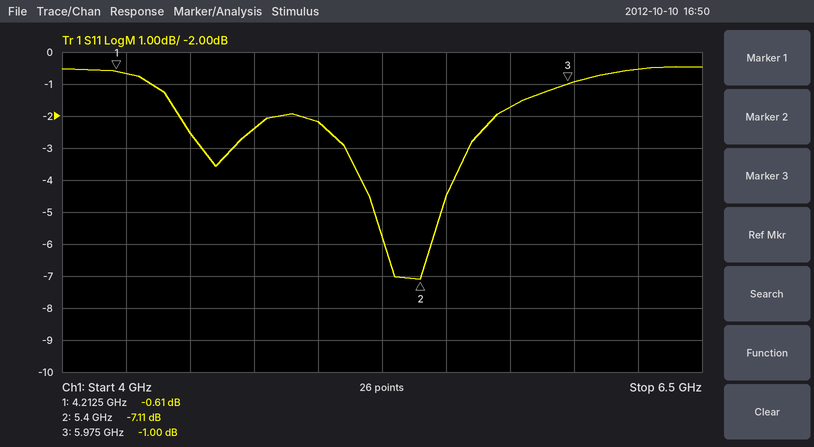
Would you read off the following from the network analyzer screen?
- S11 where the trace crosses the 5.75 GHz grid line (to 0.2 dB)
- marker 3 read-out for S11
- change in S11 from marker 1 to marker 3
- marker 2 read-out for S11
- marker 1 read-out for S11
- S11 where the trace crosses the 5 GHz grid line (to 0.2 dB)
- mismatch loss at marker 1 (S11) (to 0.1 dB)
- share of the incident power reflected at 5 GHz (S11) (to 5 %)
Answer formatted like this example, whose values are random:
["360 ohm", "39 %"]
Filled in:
["-1.8 dB", "-1.00 dB", "-0.39 dB", "-7.11 dB", "-0.61 dB", "-2.2 dB", "8.8 dB", "60 %"]
